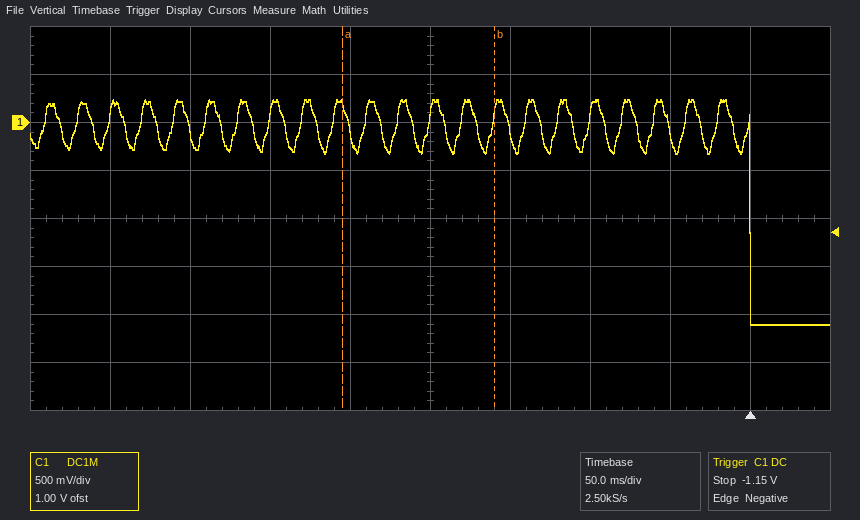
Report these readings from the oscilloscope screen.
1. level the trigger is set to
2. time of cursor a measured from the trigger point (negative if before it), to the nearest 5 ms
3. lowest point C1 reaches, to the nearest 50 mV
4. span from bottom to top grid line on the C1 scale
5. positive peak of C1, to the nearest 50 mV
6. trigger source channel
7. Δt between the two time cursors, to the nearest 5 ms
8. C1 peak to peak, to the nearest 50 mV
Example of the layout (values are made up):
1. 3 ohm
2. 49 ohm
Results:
1. -1.15 V
2. -255 ms
3. -2.10 V
4. 4 V
5. 250 mV
6. C1
7. 95 ms
8. 2.35 V
